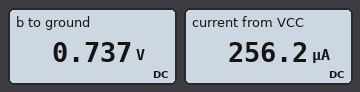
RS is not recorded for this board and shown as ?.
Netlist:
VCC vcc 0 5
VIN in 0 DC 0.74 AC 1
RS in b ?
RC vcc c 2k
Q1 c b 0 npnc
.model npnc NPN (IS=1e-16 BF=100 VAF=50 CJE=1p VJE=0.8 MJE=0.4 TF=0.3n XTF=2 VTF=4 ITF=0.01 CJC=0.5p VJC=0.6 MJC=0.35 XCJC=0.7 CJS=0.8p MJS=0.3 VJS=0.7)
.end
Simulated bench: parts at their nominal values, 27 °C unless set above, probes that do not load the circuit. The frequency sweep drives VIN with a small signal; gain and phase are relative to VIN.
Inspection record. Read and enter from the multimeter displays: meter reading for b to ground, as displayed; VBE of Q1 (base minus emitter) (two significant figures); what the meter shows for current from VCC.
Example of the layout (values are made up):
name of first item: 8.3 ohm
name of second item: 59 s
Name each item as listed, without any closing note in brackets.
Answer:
meter reading for b to ground, as displayed: 0.737 V
VBE of Q1 (base minus emitter): 740 mV
what the meter shows for current from VCC: 256.2 µA
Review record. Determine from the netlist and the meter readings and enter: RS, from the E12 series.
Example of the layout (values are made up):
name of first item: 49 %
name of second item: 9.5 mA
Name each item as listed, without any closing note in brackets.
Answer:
RS, from the E12 series: 1.2 kΩ
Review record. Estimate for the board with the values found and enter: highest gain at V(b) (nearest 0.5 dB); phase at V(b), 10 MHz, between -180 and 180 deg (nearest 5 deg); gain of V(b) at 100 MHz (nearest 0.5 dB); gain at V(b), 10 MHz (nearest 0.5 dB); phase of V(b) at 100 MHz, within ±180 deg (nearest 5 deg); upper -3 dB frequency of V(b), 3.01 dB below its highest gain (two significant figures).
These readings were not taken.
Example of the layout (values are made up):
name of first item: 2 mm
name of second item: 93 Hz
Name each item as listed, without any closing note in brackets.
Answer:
highest gain at V(b): -1.0 dB
phase at V(b), 10 MHz, between -180 and 180 deg: -35 deg
gain of V(b) at 100 MHz: -16.5 dB
gain at V(b), 10 MHz: -2.5 dB
phase of V(b) at 100 MHz, within ±180 deg: -65 deg
upper -3 dB frequency of V(b), 3.01 dB below its highest gain: 14 MHz
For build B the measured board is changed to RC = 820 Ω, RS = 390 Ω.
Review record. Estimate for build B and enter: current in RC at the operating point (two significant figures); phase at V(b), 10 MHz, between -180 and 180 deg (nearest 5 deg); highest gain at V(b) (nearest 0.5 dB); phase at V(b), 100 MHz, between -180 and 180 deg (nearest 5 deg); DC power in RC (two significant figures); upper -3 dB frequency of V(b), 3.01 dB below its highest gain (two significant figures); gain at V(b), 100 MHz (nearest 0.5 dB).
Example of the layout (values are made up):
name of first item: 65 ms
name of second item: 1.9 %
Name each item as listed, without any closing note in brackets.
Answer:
current in RC at the operating point: 280 µA
phase at V(b), 10 MHz, between -180 and 180 deg: -10 deg
highest gain at V(b): -0.5 dB
phase at V(b), 100 MHz, between -180 and 180 deg: -55 deg
DC power in RC: 63 µW
upper -3 dB frequency of V(b), 3.01 dB below its highest gain: 55 MHz
gain at V(b), 100 MHz: -6.5 dB
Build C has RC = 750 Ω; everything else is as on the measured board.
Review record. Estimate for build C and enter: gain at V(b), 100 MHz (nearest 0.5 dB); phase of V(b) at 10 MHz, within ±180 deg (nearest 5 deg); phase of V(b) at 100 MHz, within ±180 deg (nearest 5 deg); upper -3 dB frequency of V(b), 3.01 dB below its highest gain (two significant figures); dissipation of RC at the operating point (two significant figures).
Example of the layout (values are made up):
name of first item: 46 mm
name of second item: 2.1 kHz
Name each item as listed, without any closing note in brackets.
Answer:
gain at V(b), 100 MHz: -14.5 dB
phase of V(b) at 10 MHz, within ±180 deg: -25 deg
phase of V(b) at 100 MHz, within ±180 deg: -75 deg
upper -3 dB frequency of V(b), 3.01 dB below its highest gain: 21 MHz
dissipation of RC at the operating point: 50 µW
